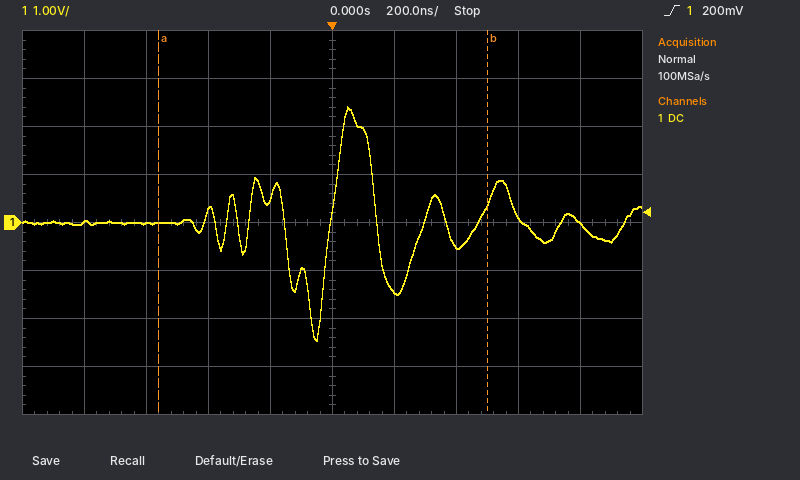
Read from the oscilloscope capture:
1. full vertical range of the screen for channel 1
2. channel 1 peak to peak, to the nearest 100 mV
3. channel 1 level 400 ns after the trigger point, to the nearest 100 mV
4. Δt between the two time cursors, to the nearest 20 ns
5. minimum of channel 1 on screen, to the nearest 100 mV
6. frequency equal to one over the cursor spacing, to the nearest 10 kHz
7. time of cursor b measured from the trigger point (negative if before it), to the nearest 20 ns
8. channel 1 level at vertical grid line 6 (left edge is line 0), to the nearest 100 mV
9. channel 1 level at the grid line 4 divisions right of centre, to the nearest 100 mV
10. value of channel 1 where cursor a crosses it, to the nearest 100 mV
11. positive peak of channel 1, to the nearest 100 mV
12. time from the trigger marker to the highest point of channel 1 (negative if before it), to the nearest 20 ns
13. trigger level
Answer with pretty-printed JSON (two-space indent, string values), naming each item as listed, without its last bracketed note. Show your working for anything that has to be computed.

{
  "full vertical range of the screen for channel 1": "8 V",
  "channel 1 peak to peak, to the nearest 100 mV": "2.4 V − (-2.5 V) = 4.9 V",
  "channel 1 level 400 ns after the trigger point, to the nearest 100 mV": "-500 mV",
  "Δt between the two time cursors, to the nearest 20 ns": "1.06 µs",
  "minimum of channel 1 on screen, to the nearest 100 mV": "-2.5 V",
  "frequency equal to one over the cursor spacing, to the nearest 10 kHz": "1 / 1.06 µs ≈ 940 kHz",
  "time of cursor b measured from the trigger point (negative if before it), to the nearest 20 ns": "+500 ns",
  "channel 1 level at vertical grid line 6 (left edge is line 0), to the nearest 100 mV": "-1.4 V",
  "channel 1 level at the grid line 4 divisions right of centre, to the nearest 100 mV": "0.0 V",
  "value of channel 1 where cursor a crosses it, to the nearest 100 mV": "0.0 V",
  "positive peak of channel 1, to the nearest 100 mV": "2.4 V",
  "time from the trigger marker to the highest point of channel 1 (negative if before it), to the nearest 20 ns": "+60 ns",
  "trigger level": "200 mV"
}
